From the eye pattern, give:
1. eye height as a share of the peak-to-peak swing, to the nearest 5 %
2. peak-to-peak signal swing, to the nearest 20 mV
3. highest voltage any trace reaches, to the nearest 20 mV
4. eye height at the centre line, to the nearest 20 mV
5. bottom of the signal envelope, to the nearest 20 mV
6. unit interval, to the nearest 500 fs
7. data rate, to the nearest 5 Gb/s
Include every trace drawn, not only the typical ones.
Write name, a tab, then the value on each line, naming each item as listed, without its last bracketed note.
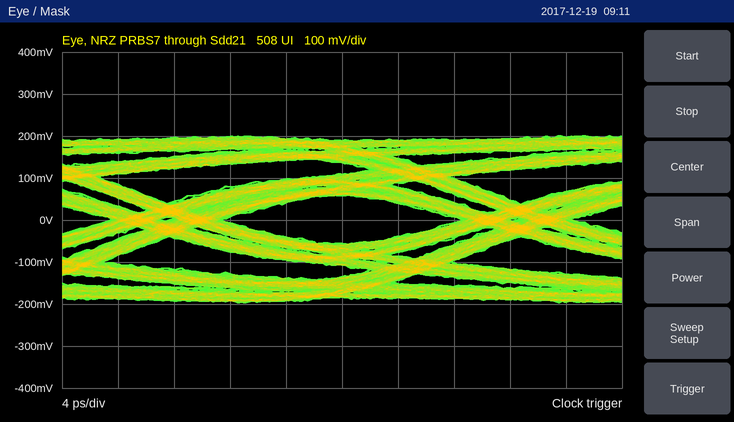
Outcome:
eye height as a share of the peak-to-peak swing, to the nearest 5 %	30 %
peak-to-peak signal swing, to the nearest 20 mV	400 mV
highest voltage any trace reaches, to the nearest 20 mV	200 mV
eye height at the centre line, to the nearest 20 mV	120 mV
bottom of the signal envelope, to the nearest 20 mV	-200 mV
unit interval, to the nearest 500 fs	25.0 ps
data rate, to the nearest 5 Gb/s	40 Gb/s
